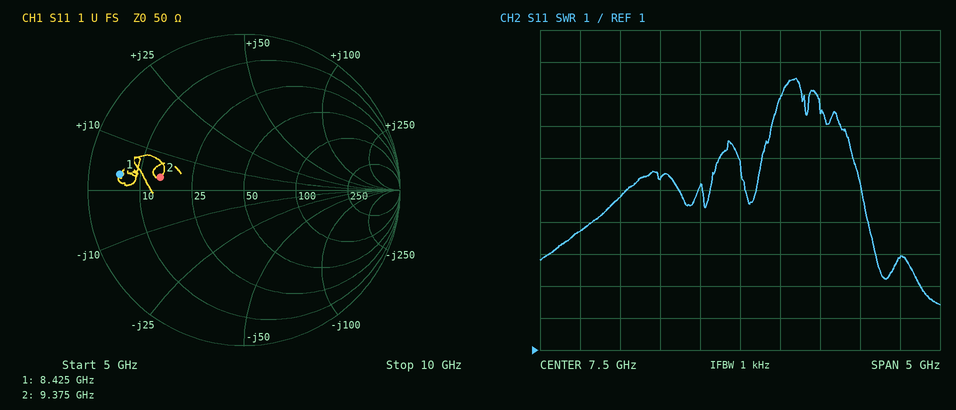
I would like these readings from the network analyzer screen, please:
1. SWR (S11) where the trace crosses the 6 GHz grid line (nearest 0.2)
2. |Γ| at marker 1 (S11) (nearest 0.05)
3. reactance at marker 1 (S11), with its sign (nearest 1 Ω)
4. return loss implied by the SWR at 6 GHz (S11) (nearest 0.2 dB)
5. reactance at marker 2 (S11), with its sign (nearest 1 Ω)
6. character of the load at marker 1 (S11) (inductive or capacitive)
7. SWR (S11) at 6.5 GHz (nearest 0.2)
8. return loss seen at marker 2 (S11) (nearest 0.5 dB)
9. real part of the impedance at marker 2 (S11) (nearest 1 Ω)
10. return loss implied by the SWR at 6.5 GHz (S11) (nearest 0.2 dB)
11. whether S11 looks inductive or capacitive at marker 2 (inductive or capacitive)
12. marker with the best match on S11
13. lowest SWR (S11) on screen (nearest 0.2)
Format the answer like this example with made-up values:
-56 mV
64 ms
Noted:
5.8
0.80
+3 Ω
3.0 dB
+3 Ω
inductive
6.4
5.5 dB
15 Ω
2.8 dB
inductive
marker 2
2.4
